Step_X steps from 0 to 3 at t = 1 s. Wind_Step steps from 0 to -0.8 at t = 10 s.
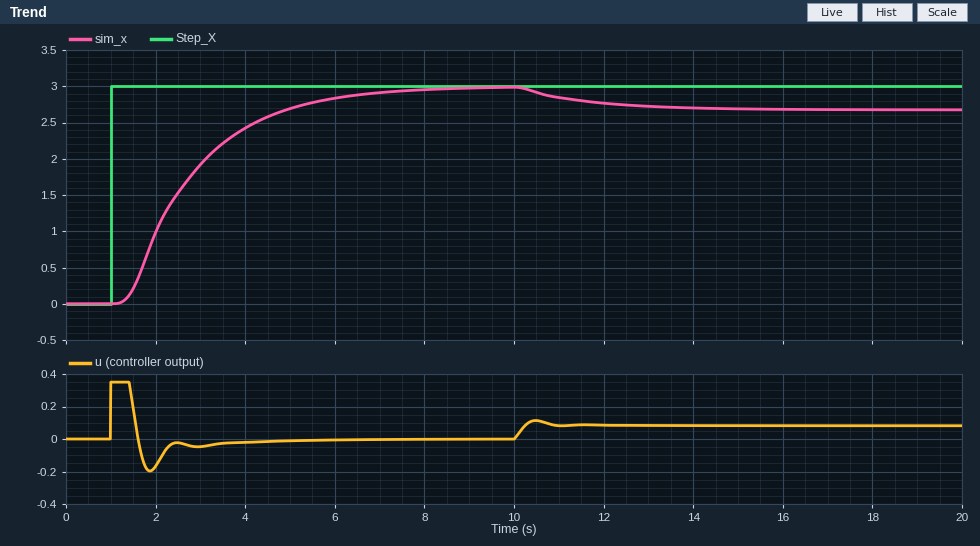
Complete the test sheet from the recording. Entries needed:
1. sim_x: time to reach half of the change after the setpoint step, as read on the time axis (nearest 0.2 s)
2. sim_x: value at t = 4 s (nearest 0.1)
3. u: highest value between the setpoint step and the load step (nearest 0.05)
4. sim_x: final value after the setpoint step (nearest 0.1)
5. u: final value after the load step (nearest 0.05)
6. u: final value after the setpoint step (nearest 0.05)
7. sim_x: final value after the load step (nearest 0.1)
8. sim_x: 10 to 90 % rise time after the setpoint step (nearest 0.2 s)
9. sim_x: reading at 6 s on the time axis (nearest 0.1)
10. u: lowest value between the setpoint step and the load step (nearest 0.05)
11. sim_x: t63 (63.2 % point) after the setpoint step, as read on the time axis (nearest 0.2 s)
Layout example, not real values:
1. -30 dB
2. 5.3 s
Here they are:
1. 2.4 s
2. 2.4
3. 0.35
4. 3.0
5. 0.10
6. 0.00
7. 2.7
8. 3.4 s
9. 2.8
10. -0.20
11. 3.0 s
